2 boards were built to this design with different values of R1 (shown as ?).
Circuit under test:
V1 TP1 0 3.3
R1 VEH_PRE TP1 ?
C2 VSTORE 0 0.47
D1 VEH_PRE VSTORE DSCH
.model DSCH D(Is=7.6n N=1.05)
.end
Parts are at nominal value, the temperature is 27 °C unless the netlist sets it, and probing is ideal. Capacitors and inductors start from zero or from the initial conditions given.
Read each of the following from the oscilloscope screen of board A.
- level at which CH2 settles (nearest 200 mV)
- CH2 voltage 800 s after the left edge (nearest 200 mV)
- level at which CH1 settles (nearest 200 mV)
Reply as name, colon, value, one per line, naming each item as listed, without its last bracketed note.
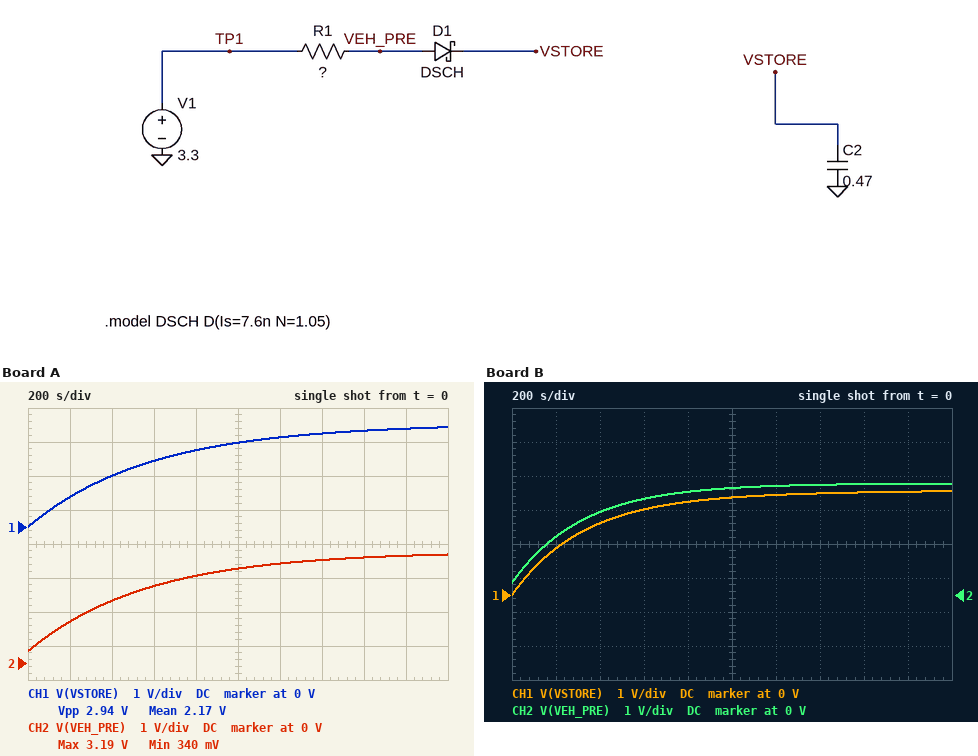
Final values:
level at which CH2 settles: 3.2 V
CH2 voltage 800 s after the left edge: 2.6 V
level at which CH1 settles: 3.0 V
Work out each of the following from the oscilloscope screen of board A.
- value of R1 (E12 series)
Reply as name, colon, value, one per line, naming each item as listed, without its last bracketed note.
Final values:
value of R1: 1.2 kΩ
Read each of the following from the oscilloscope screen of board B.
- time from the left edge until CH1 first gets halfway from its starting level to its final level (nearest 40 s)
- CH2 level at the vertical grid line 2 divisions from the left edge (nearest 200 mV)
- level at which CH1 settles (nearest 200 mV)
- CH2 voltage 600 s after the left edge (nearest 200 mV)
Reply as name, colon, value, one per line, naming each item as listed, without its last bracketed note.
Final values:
time from the left edge until CH1 first gets halfway from its starting level to its final level: 240 s
CH2 level at the vertical grid line 2 divisions from the left edge: 2.4 V
level at which CH1 settles: 3.0 V
CH2 voltage 600 s after the left edge: 2.8 V
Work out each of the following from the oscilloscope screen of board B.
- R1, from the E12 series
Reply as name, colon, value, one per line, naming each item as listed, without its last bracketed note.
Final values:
R1, from the E12 series: 680 Ω
